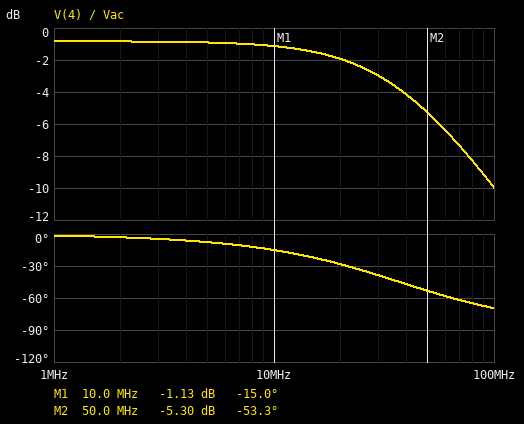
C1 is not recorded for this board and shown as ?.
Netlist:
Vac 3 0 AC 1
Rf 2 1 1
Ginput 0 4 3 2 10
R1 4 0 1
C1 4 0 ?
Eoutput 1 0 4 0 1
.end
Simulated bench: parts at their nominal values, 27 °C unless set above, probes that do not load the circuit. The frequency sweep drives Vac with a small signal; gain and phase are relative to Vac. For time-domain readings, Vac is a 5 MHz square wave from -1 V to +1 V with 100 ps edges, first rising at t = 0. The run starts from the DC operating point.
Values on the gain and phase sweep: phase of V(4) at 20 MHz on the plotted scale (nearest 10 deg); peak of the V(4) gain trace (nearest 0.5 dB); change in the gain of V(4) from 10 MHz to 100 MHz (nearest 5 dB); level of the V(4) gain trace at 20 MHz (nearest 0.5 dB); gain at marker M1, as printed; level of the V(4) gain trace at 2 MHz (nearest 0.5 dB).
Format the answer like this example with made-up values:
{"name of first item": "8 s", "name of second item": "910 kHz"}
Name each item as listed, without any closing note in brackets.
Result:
{"phase of V(4) at 20 MHz on the plotted scale": "-30 deg", "peak of the V(4) gain trace": "-1.0 dB", "change in the gain of V(4) from 10 MHz to 100 MHz": "-10 dB", "level of the V(4) gain trace at 20 MHz": "-2.0 dB", "gain at marker M1, as printed": "-1.13 dB", "level of the V(4) gain trace at 2 MHz": "-1.0 dB"}
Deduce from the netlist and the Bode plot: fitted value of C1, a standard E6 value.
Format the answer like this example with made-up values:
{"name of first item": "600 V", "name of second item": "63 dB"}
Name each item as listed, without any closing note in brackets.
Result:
{"fitted value of C1, a standard E6 value": "47 nF"}
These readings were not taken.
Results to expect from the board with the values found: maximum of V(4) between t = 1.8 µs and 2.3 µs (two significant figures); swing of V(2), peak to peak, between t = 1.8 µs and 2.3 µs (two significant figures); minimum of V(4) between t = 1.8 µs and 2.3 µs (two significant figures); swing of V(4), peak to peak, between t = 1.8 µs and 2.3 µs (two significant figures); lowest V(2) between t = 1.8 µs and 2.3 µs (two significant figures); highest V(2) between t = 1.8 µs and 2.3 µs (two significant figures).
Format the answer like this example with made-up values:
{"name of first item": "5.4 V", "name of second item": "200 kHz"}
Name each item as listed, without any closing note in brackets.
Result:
{"maximum of V(4) between t = 1.8 µs and 2.3 µs": "910 mV", "swing of V(2), peak to peak, between t = 1.8 µs and 2.3 µs": "1.8 V", "minimum of V(4) between t = 1.8 µs and 2.3 µs": "-910 mV", "swing of V(4), peak to peak, between t = 1.8 µs and 2.3 µs": "1.8 V", "lowest V(2) between t = 1.8 µs and 2.3 µs": "-910 mV", "highest V(2) between t = 1.8 µs and 2.3 µs": "910 mV"}
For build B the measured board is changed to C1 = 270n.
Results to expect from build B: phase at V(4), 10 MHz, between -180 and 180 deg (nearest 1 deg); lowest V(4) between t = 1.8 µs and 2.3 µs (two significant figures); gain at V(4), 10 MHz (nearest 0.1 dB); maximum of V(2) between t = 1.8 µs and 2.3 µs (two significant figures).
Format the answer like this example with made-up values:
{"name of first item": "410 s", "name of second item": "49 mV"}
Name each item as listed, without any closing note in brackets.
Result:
{"phase at V(4), 10 MHz, between -180 and 180 deg": "-57 deg", "lowest V(4) between t = 1.8 µs and 2.3 µs": "-880 mV", "gain at V(4), 10 MHz": "-6.1 dB", "maximum of V(2) between t = 1.8 µs and 2.3 µs": "880 mV"}
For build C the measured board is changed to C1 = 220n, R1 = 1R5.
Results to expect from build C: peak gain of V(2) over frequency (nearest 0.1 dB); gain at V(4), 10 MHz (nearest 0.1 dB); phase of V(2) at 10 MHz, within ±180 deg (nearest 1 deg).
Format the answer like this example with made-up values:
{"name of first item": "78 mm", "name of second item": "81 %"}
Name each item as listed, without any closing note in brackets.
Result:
{"peak gain of V(2) over frequency": "-0.6 dB", "gain at V(4), 10 MHz": "-4.8 dB", "phase of V(2) at 10 MHz, within ±180 deg": "-52 deg"}
